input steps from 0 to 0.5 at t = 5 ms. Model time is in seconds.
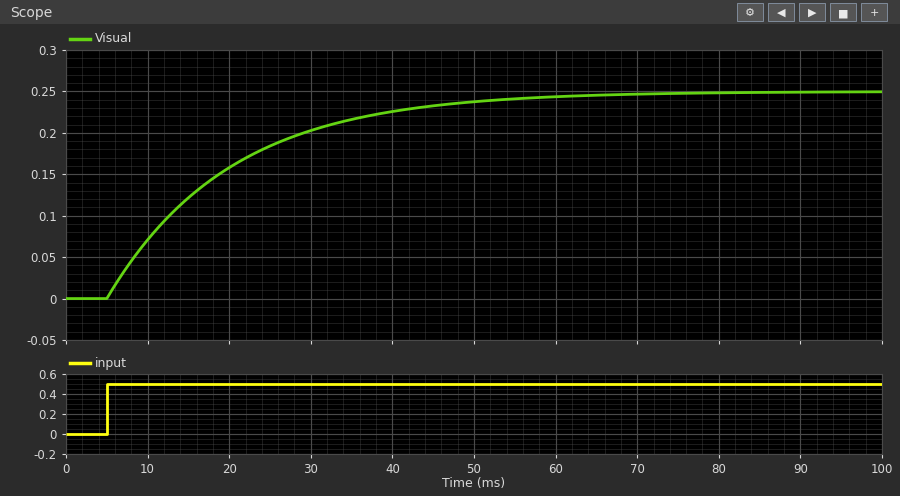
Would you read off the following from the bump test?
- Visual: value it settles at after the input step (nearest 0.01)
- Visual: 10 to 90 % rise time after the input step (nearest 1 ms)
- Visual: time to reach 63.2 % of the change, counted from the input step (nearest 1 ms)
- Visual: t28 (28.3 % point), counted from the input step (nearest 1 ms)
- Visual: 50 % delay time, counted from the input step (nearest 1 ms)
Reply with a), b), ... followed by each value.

a) 0.25
b) 33 ms
c) 15 ms
d) 5 ms
e) 10 ms
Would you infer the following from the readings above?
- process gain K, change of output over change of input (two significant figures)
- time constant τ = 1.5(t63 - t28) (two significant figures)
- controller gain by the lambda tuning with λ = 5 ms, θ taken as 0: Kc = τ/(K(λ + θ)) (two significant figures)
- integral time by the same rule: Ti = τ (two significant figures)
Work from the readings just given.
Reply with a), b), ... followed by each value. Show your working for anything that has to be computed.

a) (0.25 - 0) / 0.5 = 0.50
b) 1.5 × (15 - 5) = 15 ms
c) 15 / (0.5 × (5 + 0)) = 6.0
d) 15 ms
